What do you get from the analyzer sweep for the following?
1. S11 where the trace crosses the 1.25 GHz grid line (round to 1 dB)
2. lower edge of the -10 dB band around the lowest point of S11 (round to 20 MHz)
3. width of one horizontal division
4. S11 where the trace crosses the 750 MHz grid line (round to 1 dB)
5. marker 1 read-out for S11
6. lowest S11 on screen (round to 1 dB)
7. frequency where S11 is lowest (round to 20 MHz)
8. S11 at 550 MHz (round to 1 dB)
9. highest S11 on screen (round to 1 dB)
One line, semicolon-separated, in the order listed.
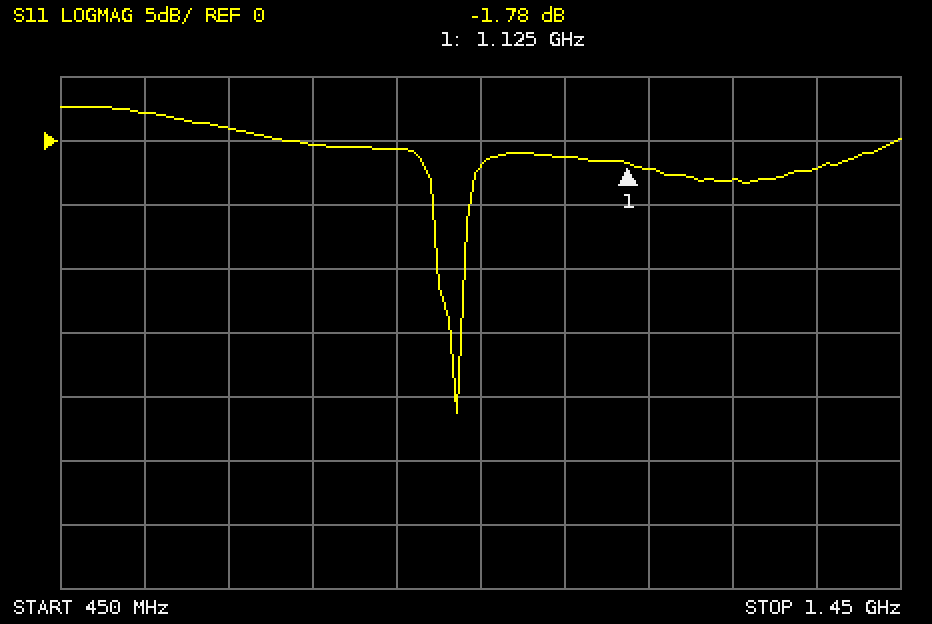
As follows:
-3 dB; 900 MHz; 100 MHz; 0 dB; -1.78 dB; -21 dB; 920 MHz; 2 dB; 3 dB
